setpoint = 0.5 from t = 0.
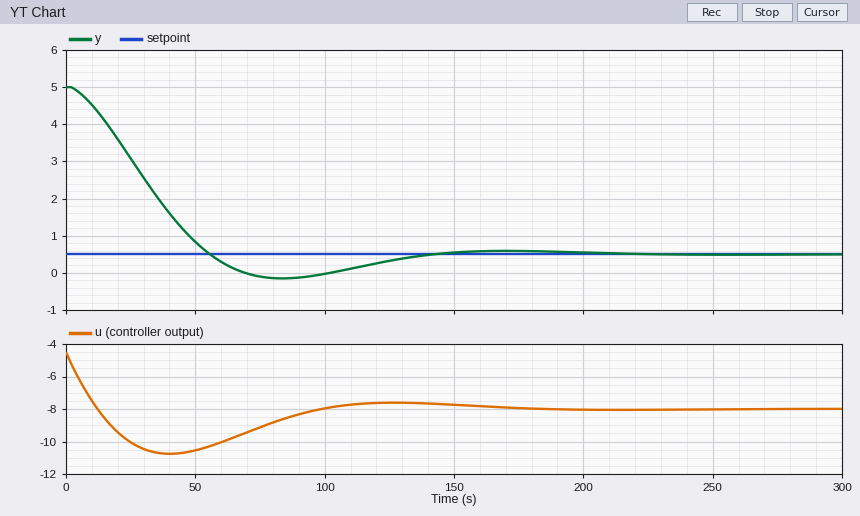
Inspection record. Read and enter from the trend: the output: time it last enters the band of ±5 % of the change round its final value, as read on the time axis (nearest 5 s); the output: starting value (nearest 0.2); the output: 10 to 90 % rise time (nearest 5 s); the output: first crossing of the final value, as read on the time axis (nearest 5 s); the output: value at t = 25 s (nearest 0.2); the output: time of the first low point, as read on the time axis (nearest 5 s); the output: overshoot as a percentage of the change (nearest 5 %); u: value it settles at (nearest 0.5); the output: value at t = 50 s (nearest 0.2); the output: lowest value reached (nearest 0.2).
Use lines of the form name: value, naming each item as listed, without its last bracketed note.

the output: time it last enters the band of ±5 % of the change round its final value, as read on the time axis: 120 s
the output: starting value: 5.0
the output: 10 to 90 % rise time: 40 s
the output: first crossing of the final value, as read on the time axis: 55 s
the output: value at t = 25 s: 3.0
the output: time of the first low point, as read on the time axis: 85 s
the output: overshoot as a percentage of the change: 15 %
u: value it settles at: -8.0
the output: value at t = 50 s: 0.8
the output: lowest value reached: -0.2
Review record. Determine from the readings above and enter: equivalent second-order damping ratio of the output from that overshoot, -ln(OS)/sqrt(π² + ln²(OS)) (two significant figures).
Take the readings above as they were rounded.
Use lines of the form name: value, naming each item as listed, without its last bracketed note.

equivalent second-order damping ratio of the output from that overshoot, -ln(OS)/sqrt(π² + ln²(OS)): 0.52
